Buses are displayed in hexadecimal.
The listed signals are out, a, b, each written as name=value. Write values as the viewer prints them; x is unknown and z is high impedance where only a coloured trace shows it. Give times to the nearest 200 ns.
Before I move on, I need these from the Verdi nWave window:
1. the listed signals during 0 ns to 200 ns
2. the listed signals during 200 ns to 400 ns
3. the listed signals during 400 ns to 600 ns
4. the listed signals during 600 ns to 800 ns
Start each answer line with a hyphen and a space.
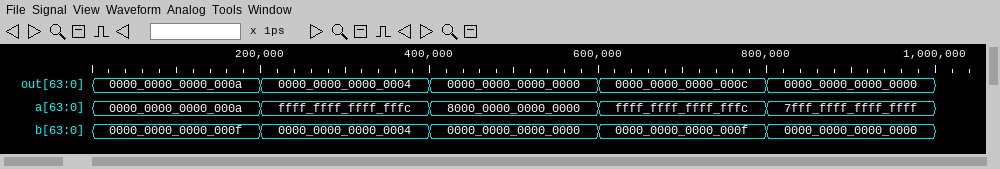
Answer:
- out=0000_0000_0000_000a, a=0000_0000_0000_000a, b=0000_0000_0000_000f
- out=0000_0000_0000_0004, a=ffff_ffff_ffff_fffc, b=0000_0000_0000_0004
- out=0000_0000_0000_0000, a=8000_0000_0000_0000, b=0000_0000_0000_0000
- out=0000_0000_0000_000c, a=ffff_ffff_ffff_fffc, b=0000_0000_0000_000f
